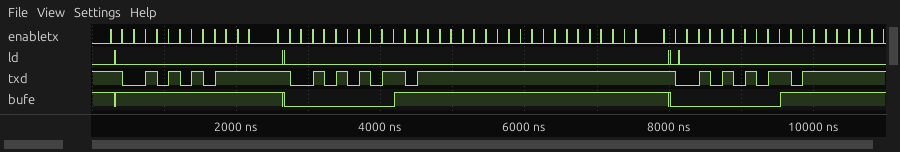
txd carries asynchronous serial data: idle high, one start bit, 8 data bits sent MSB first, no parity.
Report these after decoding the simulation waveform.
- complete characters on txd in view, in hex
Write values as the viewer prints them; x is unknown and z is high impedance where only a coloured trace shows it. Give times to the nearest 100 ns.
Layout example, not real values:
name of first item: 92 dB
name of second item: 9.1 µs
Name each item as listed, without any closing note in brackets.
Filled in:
complete characters on txd in view, in hex: 55, 55, FF, 55
